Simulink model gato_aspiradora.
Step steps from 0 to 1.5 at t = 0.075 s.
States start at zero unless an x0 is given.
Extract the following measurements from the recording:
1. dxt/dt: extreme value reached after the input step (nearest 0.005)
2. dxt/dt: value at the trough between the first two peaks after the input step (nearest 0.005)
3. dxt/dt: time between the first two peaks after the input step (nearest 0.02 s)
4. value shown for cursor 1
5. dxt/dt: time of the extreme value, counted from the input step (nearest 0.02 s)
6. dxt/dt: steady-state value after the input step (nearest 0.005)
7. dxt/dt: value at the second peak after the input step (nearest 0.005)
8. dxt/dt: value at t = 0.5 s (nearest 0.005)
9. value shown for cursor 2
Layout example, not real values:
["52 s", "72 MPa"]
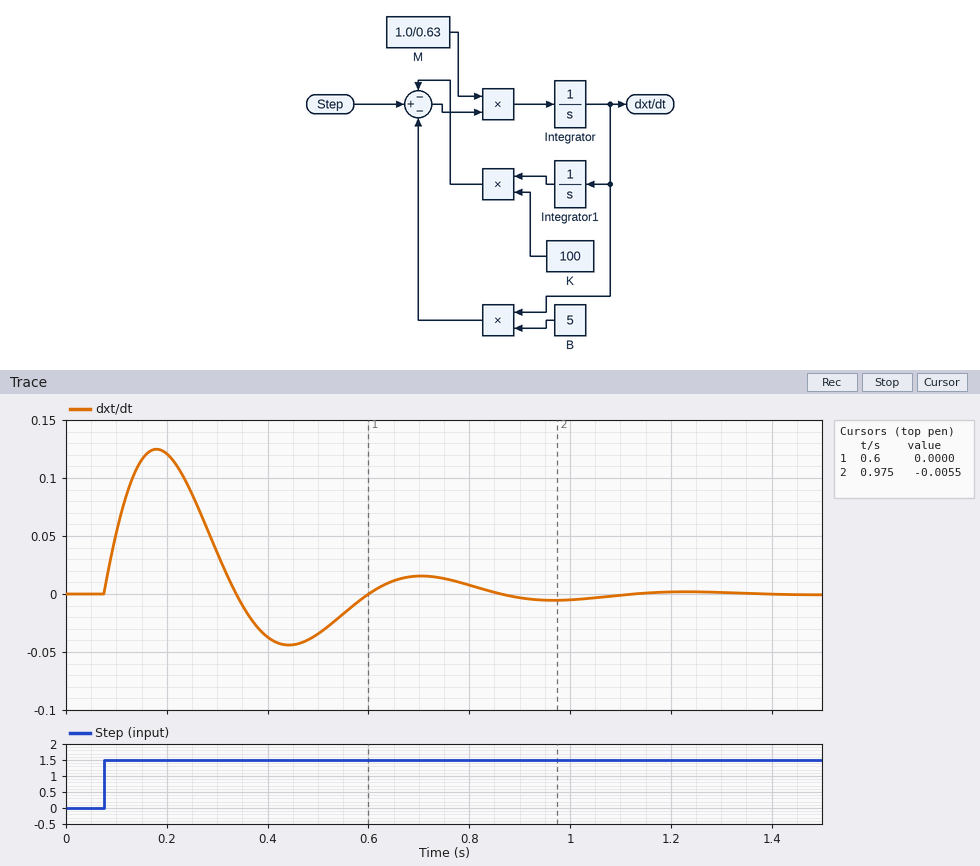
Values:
["0.125", "-0.045", "0.52 s", "0.0000", "0.10 s", "0.000", "0.015", "-0.035", "-0.0055"]
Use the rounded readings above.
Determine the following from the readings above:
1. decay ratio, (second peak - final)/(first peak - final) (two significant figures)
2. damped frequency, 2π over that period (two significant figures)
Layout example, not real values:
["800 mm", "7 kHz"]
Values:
["0.12", "12 rad/s"]
